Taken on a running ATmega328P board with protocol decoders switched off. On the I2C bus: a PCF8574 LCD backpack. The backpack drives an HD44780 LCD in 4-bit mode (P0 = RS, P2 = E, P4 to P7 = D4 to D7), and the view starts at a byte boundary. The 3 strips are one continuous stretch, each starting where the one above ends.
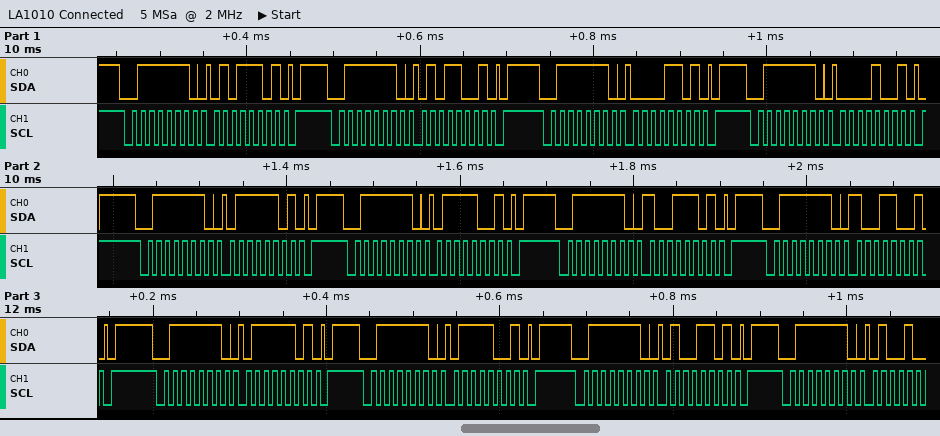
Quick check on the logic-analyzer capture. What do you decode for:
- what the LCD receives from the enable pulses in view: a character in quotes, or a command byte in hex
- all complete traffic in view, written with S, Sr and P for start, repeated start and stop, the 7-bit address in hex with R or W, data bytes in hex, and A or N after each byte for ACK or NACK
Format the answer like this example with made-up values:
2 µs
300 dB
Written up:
'P' 'y'
S 3FW A 5D A P S 3FW A 59 A P S 3FW A 0D A P S 3FW A 09 A P S 3FW A 7D A P S 3FW A 79 A P S 3FW A 9D A P S 3FW A 99 A P S 3FW A 7D A P S 3FW A 79 A P S 3FW A 4D A P S 3FW A
